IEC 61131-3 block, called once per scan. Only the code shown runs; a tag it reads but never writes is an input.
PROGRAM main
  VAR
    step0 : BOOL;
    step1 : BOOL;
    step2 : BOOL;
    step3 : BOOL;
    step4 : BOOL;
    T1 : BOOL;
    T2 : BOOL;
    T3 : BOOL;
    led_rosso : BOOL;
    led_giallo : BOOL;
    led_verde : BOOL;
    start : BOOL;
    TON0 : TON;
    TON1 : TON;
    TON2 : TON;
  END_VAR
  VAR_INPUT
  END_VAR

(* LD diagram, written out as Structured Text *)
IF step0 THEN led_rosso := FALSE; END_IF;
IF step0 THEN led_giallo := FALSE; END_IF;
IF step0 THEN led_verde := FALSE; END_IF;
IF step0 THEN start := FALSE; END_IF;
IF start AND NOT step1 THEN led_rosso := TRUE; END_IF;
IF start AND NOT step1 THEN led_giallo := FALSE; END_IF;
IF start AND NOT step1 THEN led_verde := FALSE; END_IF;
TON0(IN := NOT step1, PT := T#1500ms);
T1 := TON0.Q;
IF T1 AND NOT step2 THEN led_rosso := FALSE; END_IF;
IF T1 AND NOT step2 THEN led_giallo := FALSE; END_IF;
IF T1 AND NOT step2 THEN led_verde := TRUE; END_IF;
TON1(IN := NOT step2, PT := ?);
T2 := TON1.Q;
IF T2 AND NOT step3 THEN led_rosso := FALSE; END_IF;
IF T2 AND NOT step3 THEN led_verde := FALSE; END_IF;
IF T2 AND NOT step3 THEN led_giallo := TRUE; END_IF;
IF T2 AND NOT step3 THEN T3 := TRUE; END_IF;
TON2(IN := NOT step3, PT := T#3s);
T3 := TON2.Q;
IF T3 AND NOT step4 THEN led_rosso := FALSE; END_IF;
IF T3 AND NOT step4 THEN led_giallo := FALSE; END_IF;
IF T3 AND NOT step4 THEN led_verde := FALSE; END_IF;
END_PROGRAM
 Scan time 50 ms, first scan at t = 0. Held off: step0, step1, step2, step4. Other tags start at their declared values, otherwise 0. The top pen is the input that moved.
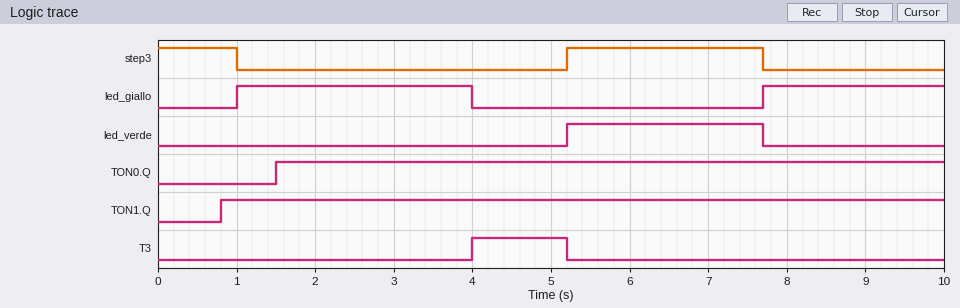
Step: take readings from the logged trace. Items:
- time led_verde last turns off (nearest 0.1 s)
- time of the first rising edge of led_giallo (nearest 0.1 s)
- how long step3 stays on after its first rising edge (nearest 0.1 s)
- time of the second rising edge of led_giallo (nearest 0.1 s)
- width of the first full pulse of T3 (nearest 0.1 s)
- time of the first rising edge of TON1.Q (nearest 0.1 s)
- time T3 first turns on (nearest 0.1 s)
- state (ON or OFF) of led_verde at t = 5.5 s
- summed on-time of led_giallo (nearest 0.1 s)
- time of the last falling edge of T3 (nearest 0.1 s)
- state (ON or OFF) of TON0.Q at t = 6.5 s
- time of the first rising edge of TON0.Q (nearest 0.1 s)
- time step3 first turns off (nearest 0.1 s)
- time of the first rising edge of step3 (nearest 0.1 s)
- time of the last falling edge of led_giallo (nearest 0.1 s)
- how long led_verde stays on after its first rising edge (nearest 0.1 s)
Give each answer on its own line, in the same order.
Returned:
7.7 s
1.0 s
2.5 s
7.7 s
1.2 s
0.8 s
4.0 s
ON
5.3 s
5.2 s
ON
1.5 s
1.0 s
5.2 s
4.0 s
2.5 s
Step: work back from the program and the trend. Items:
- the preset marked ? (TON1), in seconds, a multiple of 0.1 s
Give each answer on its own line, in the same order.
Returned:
0.8 s
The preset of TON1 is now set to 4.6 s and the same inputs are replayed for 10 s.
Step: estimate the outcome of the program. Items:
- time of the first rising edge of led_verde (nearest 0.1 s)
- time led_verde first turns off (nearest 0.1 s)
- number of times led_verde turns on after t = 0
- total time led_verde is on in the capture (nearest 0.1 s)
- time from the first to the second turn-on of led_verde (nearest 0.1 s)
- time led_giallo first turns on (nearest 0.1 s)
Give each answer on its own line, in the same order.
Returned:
1.5 s
4.0 s
2
5.0 s
3.7 s
7.7 s
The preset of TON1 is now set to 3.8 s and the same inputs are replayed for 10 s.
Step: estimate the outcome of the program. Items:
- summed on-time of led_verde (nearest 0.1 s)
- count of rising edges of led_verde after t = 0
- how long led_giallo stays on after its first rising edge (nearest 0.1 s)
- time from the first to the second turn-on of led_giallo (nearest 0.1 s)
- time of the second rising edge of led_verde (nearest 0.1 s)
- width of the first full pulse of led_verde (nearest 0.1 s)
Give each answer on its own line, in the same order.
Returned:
4.8 s
2
0.2 s
3.9 s
5.2 s
2.3 s
